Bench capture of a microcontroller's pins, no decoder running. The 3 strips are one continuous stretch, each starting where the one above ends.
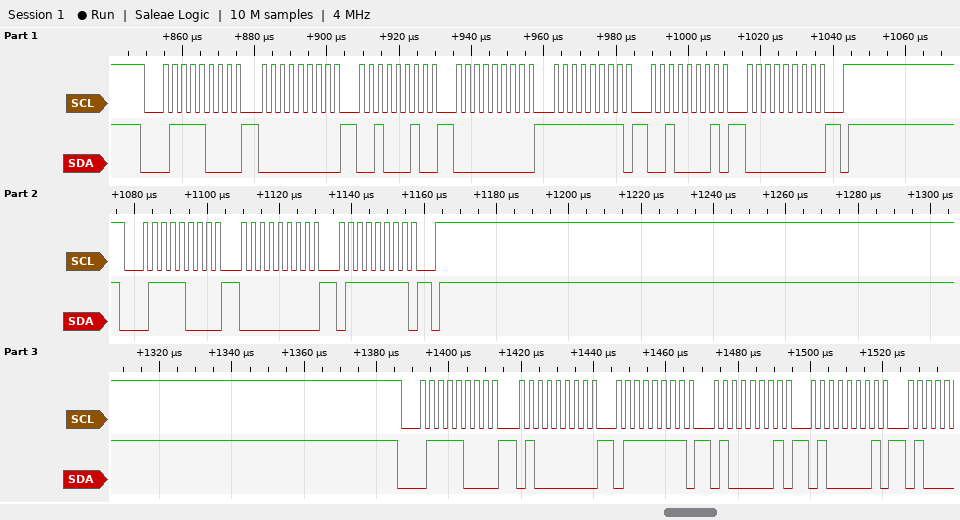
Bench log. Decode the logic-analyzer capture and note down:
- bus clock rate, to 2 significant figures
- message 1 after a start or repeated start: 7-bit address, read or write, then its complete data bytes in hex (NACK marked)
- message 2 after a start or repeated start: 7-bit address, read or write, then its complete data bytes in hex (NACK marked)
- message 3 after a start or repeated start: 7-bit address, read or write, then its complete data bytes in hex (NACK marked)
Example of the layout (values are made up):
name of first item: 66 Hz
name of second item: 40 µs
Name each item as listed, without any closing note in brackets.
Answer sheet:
bus clock rate, to 2 significant figures: 400 kHz
message 1 after a start or repeated start: 7-bit address, read or write, then its complete data bytes in hex: 0x3C write: 00 22 00 FF 21 00
message 2 after a start or repeated start: 7-bit address, read or write, then its complete data bytes in hex: 0x3C write: 00 7F
message 3 after a start or repeated start: 7-bit address, read or write, then its complete data bytes in hex: 0x3C write: 40 7F 41 41
